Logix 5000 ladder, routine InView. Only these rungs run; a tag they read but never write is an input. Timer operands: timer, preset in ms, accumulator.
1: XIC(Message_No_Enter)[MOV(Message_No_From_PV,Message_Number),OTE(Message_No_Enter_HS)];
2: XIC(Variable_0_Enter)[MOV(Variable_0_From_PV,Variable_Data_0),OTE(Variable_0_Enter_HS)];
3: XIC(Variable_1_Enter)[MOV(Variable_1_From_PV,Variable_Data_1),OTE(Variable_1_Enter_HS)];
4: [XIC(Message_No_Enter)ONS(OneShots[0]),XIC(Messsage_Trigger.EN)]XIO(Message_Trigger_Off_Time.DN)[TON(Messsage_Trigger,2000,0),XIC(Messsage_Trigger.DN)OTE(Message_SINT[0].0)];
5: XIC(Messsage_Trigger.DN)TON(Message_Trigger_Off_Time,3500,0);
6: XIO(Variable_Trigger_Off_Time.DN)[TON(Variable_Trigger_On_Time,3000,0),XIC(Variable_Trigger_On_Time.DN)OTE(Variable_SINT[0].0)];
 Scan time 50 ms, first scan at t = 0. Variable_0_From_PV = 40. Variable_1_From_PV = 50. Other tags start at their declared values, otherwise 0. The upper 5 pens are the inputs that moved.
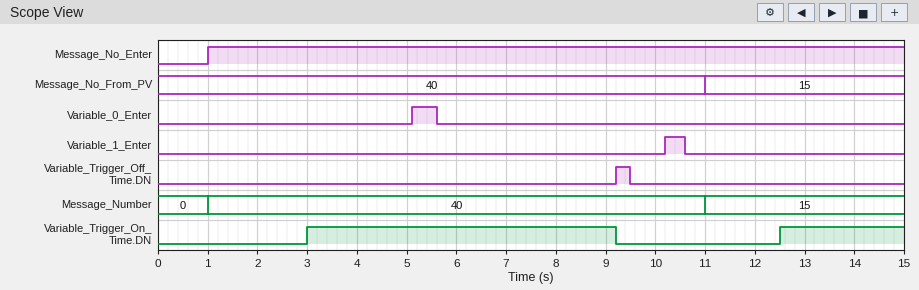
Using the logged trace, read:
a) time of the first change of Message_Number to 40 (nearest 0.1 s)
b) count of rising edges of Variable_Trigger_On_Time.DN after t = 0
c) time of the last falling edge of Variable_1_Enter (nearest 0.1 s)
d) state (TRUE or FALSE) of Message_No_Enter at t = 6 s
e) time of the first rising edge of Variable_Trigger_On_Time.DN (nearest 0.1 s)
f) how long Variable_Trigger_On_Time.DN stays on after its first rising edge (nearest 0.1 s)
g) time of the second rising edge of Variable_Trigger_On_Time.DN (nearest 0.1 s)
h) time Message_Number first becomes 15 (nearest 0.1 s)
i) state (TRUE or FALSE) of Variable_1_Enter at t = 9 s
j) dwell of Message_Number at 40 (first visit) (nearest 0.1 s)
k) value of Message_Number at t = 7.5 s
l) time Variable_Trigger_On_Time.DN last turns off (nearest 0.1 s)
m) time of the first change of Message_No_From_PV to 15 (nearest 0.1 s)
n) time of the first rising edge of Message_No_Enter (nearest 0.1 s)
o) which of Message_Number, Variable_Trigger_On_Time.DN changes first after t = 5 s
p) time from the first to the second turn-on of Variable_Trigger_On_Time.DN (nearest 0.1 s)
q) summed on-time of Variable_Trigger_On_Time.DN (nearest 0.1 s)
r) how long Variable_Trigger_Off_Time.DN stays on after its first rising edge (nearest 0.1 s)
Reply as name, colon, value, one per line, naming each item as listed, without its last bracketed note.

time of the first change of Message_Number to 40: 1.0 s
count of rising edges of Variable_Trigger_On_Time.DN after t = 0: 2
time of the last falling edge of Variable_1_Enter: 10.6 s
state (TRUE or FALSE) of Message_No_Enter at t = 6 s: TRUE
time of the first rising edge of Variable_Trigger_On_Time.DN: 3.0 s
how long Variable_Trigger_On_Time.DN stays on after its first rising edge: 6.2 s
time of the second rising edge of Variable_Trigger_On_Time.DN: 12.5 s
time Message_Number first becomes 15: 11.0 s
state (TRUE or FALSE) of Variable_1_Enter at t = 9 s: FALSE
dwell of Message_Number at 40 (first visit): 10.0 s
value of Message_Number at t = 7.5 s: 40
time Variable_Trigger_On_Time.DN last turns off: 9.2 s
time of the first change of Message_No_From_PV to 15: 11.0 s
time of the first rising edge of Message_No_Enter: 1.0 s
which of Message_Number, Variable_Trigger_On_Time.DN changes first after t = 5 s: Variable_Trigger_On_Time.DN
time from the first to the second turn-on of Variable_Trigger_On_Time.DN: 9.5 s
summed on-time of Variable_Trigger_On_Time.DN: 8.7 s
how long Variable_Trigger_Off_Time.DN stays on after its first rising edge: 0.3 s
